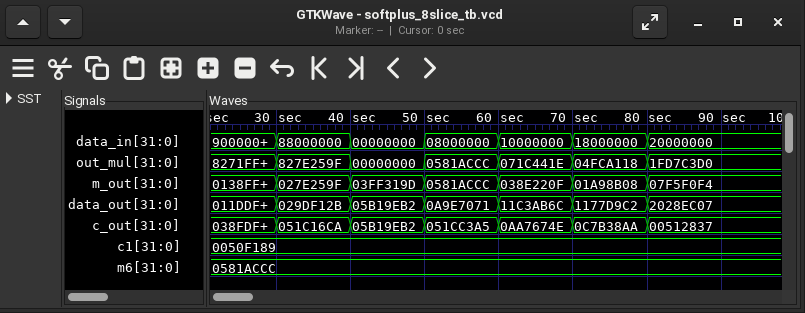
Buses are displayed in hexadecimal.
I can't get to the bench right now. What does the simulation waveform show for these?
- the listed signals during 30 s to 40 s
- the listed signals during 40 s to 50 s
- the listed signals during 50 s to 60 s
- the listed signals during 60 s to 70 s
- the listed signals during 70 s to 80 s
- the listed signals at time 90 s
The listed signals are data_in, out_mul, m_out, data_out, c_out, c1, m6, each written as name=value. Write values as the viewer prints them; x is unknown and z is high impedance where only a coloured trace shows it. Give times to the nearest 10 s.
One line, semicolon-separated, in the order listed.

data_in=88000000, out_mul=827E259F, m_out=027E259F, data_out=029DF12B, c_out=051C16CA, c1=0050F189, m6=0581ACCC; data_in=00000000, out_mul=00000000, m_out=03FF319D, data_out=05B19EB2, c_out=05B19EB2, c1=0050F189, m6=0581ACCC; data_in=08000000, out_mul=0581ACCC, m_out=0581ACCC, data_out=0A9E7071, c_out=051CC3A5, c1=0050F189, m6=0581ACCC; data_in=10000000, out_mul=071C441E, m_out=038E220F, data_out=11C3AB6C, c_out=0AA7674E, c1=0050F189, m6=0581ACCC; data_in=18000000, out_mul=04FCA118, m_out=01A98B08, data_out=1177D9C2, c_out=0C7B38AA, c1=0050F189, m6=0581ACCC; data_in=20000000, out_mul=1FD7C3D0, m_out=07F5F0F4, data_out=2028EC07, c_out=00512837, c1=0050F189, m6=0581ACCC
